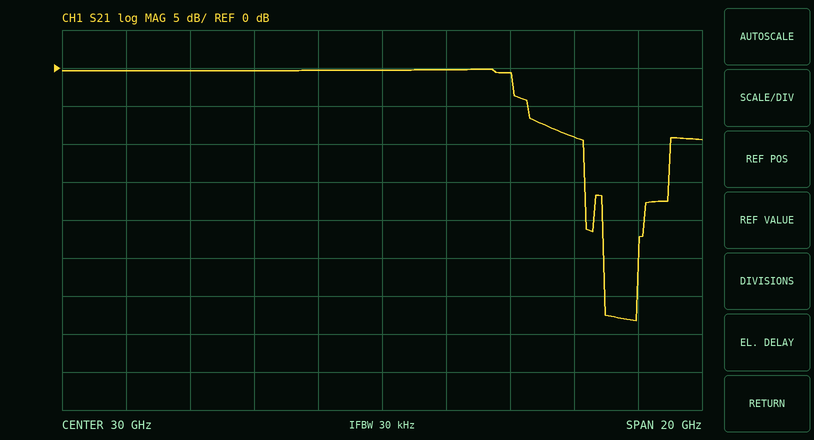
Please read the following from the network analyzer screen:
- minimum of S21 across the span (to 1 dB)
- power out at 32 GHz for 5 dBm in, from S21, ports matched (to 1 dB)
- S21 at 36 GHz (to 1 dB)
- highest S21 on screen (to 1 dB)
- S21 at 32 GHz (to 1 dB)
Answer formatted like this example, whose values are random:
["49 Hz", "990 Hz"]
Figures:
["-33 dB", "5 dBm", "-9 dB", "0 dB", "0 dB"]
